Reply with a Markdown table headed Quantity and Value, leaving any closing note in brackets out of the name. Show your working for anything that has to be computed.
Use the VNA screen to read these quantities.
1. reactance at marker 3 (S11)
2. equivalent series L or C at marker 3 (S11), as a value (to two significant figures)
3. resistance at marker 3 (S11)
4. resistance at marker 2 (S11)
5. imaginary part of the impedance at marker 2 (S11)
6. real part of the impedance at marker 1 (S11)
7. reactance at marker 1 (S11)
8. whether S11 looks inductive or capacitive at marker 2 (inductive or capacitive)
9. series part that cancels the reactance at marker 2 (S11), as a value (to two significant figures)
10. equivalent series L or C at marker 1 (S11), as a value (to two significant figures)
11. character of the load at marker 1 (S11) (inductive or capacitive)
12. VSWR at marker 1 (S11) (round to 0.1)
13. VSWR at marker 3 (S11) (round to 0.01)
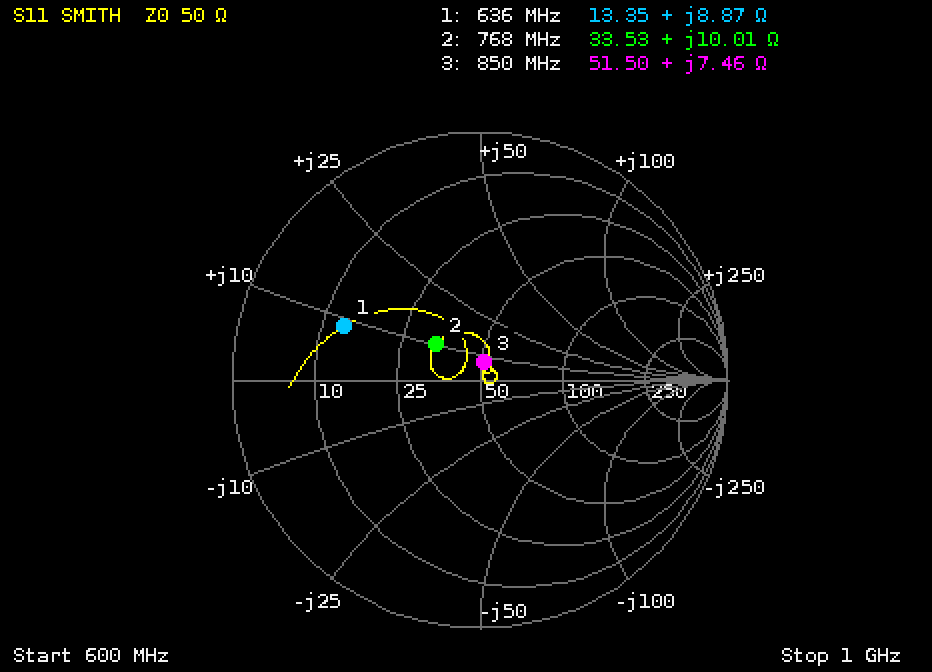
| Quantity | Value |
|---|---|
| reactance at marker 3 | +7.46 Ω |
| equivalent series L or C at marker 3 (S11), as a value | L = 7.46 Ω/(2π × 850 MHz) ≈ 1.4 nH |
| resistance at marker 3 | 51.50 Ω |
| resistance at marker 2 | 33.53 Ω |
| imaginary part of the impedance at marker 2 | +10.01 Ω |
| real part of the impedance at marker 1 | 13.35 Ω |
| reactance at marker 1 | +8.87 Ω |
| whether S11 looks inductive or capacitive at marker 2 | inductive |
| series part that cancels the reactance at marker 2 (S11), as a value | C = 1/(2π × 768 MHz × 10.01 Ω) ≈ 21 pF |
| equivalent series L or C at marker 1 (S11), as a value | L = 8.87 Ω/(2π × 636 MHz) ≈ 2.2 nH |
| character of the load at marker 1 (S11) | inductive |
| VSWR at marker 1 (S11) | 3.9 |
| VSWR at marker 3 (S11) | 1.16 |
